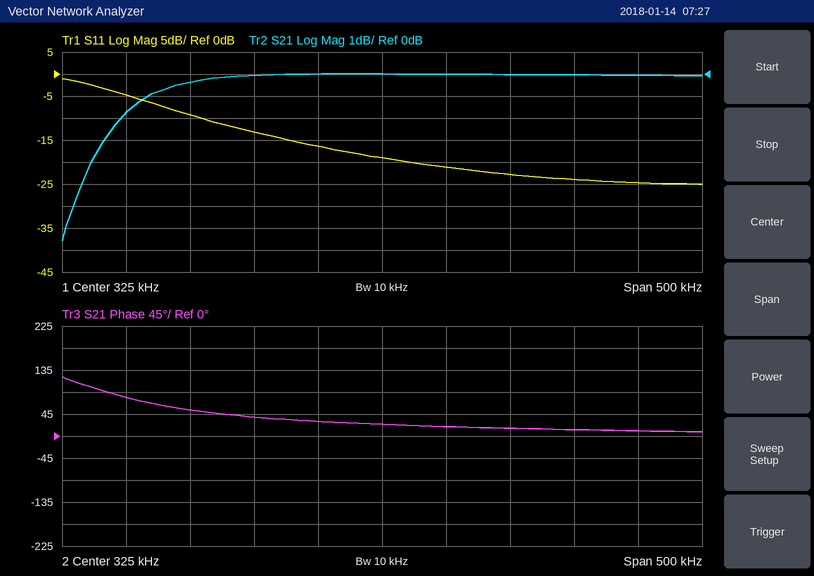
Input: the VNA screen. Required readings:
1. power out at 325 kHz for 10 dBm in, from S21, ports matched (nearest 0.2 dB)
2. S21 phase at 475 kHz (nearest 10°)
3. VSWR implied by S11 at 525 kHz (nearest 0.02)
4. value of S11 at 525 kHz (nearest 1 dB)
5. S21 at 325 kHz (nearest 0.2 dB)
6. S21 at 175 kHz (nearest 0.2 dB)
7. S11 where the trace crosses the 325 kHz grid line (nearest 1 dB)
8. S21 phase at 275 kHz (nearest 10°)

10.0 dBm
10°
1.12
-25 dB
0.0 dB
-0.4 dB
-19 dB
30°
